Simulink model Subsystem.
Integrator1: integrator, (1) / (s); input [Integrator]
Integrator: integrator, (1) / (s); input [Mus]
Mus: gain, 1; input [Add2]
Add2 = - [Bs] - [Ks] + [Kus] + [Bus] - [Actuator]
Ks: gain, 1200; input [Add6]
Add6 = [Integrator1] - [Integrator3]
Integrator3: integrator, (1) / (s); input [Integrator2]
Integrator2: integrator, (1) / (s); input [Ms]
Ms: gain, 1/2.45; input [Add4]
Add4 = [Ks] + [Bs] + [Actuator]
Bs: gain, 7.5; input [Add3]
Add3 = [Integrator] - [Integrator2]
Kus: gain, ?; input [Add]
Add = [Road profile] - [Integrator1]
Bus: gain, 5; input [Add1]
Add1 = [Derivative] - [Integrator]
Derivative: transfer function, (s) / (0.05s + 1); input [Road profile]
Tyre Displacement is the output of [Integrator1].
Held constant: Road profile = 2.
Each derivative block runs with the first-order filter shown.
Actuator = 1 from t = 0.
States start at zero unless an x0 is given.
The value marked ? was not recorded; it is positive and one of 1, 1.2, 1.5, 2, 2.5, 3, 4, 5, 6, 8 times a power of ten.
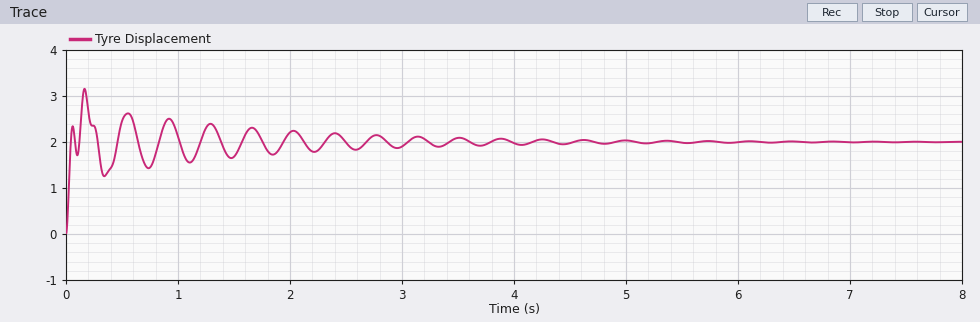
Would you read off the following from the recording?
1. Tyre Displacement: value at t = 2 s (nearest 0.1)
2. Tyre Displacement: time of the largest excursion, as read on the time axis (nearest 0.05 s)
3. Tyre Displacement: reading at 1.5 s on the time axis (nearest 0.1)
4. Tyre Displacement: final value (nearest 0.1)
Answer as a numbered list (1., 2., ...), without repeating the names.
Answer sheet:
1. 2.2
2. 0.15 s
3. 1.7
4. 2.0
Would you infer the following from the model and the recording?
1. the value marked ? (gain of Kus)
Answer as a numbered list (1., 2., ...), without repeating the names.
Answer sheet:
1. 2000
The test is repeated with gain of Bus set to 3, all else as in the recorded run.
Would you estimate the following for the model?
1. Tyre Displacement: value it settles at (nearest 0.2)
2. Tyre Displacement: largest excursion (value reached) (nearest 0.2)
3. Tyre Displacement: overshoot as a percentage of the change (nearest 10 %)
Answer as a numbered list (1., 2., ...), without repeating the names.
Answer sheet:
1. 2.0
2. 3.2
3. 60 %
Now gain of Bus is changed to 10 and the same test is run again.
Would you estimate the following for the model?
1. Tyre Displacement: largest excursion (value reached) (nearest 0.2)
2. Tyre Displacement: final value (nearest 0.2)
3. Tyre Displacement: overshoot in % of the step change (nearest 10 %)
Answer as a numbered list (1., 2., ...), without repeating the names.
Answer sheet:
1. 3.0
2. 2.0
3. 50 %
